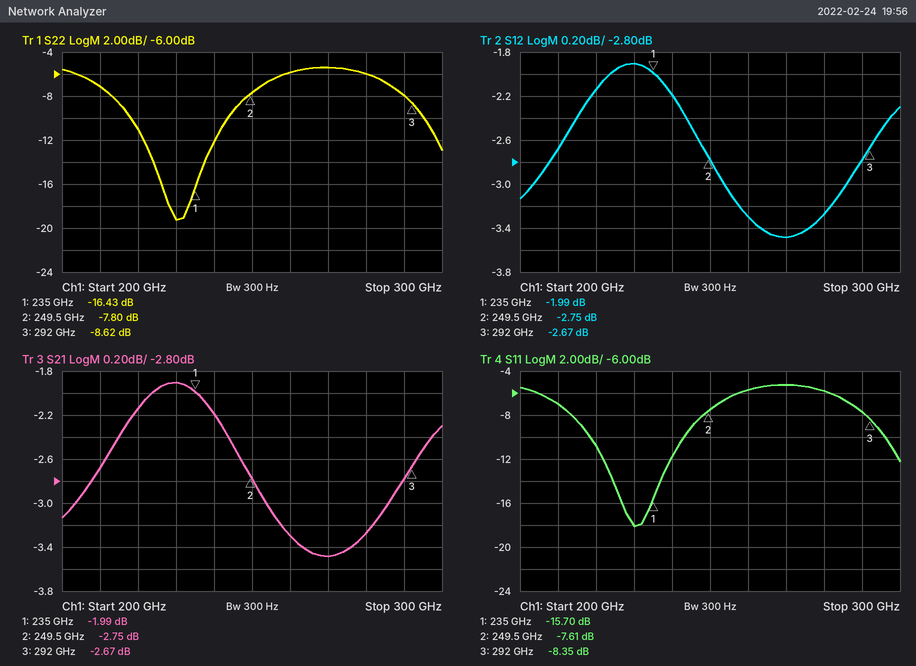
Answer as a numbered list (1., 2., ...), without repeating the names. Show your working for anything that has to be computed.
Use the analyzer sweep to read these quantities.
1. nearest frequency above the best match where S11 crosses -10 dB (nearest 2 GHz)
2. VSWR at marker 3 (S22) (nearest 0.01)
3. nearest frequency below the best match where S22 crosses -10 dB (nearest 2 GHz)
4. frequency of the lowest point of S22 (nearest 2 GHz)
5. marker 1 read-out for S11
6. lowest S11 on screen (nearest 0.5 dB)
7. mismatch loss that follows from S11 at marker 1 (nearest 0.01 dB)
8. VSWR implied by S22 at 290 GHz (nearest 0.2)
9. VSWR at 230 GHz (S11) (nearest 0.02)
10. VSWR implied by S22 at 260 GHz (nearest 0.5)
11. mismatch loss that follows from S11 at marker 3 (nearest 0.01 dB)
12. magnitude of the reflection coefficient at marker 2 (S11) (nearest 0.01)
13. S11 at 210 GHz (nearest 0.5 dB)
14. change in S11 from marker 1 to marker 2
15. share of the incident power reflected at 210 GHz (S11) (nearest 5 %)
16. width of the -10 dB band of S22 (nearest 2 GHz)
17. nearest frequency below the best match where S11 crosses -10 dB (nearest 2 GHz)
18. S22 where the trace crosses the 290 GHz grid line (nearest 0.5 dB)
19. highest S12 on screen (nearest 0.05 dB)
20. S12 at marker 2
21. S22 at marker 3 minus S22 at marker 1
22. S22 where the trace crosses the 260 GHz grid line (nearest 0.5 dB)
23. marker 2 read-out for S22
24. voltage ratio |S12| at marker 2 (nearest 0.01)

1. 244 GHz
2. (1 + 0.3707)/(1 − 0.3707) ≈ 2.18
3. 218 GHz
4. 230 GHz
5. -15.70 dB
6. -18.0 dB
7. −10 log10(1 − 10^(-15.7/10)) ≈ 0.12 dB
8. |Γ| = 10^(-8/20) = 0.3981; VSWR = (1 + 0.3981)/(1 − 0.3981) ≈ 2.32, so 2.4 to the nearest 0.2
9. |Γ| = 10^(-18/20) = 0.1259; VSWR = (1 + 0.1259)/(1 − 0.1259) ≈ 1.29, so 1.28 to the nearest 0.02
10. |Γ| = 10^(-6/20) = 0.5012; VSWR = (1 + 0.5012)/(1 − 0.5012) ≈ 3.0
11. −10 log10(1 − 10^(-8.35/10)) ≈ 0.69 dB
12. 10^(-7.61/20) ≈ 0.42
13. -7.0 dB
14. -7.61 − (-15.7) = 8.09 dB
15. 10^(-7/10) ≈ 20 %
16. 244 GHz − 218 GHz = 26 GHz
17. 218 GHz
18. -8.0 dB
19. -1.90 dB
20. -2.75 dB
21. -8.62 − (-16.43) = 7.81 dB
22. -6.0 dB
23. -7.80 dB
24. 10^(-2.75/20) ≈ 0.73
